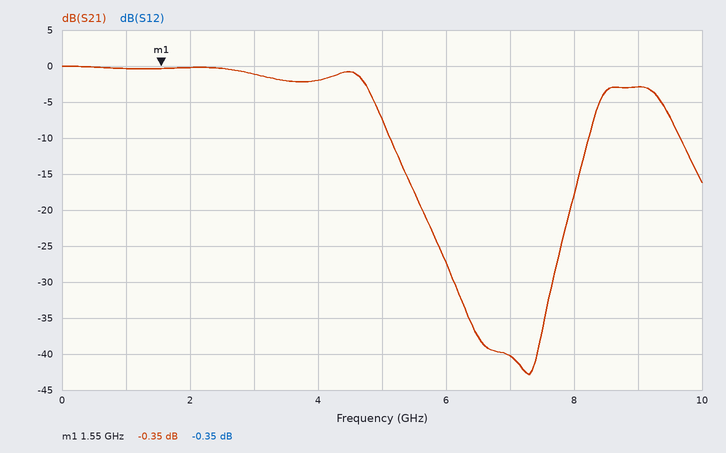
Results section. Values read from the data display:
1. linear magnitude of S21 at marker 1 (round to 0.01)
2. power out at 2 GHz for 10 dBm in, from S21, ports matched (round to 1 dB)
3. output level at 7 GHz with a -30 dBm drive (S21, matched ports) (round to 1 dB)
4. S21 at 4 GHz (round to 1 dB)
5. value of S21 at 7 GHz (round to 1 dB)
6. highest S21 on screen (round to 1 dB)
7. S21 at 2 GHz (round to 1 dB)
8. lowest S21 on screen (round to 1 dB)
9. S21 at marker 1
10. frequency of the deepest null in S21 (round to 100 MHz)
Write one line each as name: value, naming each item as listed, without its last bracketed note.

linear magnitude of S21 at marker 1: 0.96
power out at 2 GHz for 10 dBm in, from S21, ports matched: 10 dBm
output level at 7 GHz with a -30 dBm drive (S21, matched ports): -70 dBm
S21 at 4 GHz: -2 dB
value of S21 at 7 GHz: -40 dB
highest S21 on screen: 0 dB
S21 at 2 GHz: 0 dB
lowest S21 on screen: -43 dB
S21 at marker 1: -0.35 dB
frequency of the deepest null in S21: 7.3 GHz
